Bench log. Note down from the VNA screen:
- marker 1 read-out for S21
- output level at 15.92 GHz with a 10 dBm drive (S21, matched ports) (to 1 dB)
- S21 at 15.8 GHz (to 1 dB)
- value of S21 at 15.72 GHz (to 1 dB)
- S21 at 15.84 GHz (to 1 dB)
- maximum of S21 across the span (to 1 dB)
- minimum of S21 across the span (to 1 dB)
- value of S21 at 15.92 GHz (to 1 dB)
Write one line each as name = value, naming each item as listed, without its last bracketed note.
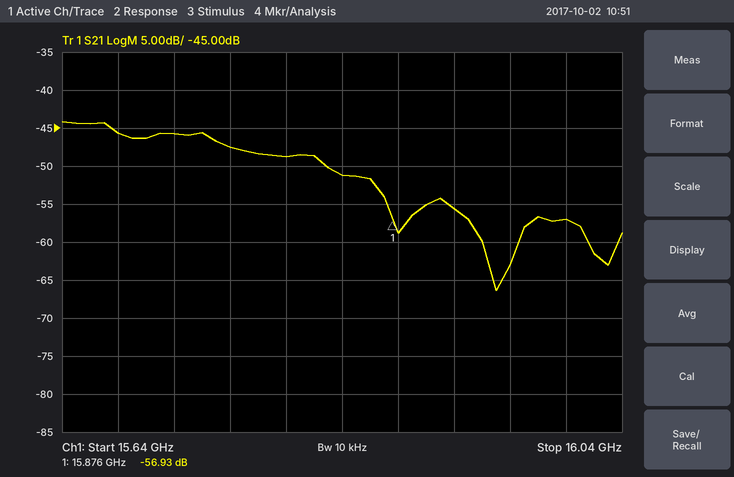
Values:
marker 1 read-out for S21 = -56.93 dB
output level at 15.92 GHz with a 10 dBm drive (S21, matched ports) = -46 dBm
S21 at 15.8 GHz = -49 dB
value of S21 at 15.72 GHz = -46 dB
S21 at 15.84 GHz = -51 dB
maximum of S21 across the span = -44 dB
minimum of S21 across the span = -66 dB
value of S21 at 15.92 GHz = -56 dB
